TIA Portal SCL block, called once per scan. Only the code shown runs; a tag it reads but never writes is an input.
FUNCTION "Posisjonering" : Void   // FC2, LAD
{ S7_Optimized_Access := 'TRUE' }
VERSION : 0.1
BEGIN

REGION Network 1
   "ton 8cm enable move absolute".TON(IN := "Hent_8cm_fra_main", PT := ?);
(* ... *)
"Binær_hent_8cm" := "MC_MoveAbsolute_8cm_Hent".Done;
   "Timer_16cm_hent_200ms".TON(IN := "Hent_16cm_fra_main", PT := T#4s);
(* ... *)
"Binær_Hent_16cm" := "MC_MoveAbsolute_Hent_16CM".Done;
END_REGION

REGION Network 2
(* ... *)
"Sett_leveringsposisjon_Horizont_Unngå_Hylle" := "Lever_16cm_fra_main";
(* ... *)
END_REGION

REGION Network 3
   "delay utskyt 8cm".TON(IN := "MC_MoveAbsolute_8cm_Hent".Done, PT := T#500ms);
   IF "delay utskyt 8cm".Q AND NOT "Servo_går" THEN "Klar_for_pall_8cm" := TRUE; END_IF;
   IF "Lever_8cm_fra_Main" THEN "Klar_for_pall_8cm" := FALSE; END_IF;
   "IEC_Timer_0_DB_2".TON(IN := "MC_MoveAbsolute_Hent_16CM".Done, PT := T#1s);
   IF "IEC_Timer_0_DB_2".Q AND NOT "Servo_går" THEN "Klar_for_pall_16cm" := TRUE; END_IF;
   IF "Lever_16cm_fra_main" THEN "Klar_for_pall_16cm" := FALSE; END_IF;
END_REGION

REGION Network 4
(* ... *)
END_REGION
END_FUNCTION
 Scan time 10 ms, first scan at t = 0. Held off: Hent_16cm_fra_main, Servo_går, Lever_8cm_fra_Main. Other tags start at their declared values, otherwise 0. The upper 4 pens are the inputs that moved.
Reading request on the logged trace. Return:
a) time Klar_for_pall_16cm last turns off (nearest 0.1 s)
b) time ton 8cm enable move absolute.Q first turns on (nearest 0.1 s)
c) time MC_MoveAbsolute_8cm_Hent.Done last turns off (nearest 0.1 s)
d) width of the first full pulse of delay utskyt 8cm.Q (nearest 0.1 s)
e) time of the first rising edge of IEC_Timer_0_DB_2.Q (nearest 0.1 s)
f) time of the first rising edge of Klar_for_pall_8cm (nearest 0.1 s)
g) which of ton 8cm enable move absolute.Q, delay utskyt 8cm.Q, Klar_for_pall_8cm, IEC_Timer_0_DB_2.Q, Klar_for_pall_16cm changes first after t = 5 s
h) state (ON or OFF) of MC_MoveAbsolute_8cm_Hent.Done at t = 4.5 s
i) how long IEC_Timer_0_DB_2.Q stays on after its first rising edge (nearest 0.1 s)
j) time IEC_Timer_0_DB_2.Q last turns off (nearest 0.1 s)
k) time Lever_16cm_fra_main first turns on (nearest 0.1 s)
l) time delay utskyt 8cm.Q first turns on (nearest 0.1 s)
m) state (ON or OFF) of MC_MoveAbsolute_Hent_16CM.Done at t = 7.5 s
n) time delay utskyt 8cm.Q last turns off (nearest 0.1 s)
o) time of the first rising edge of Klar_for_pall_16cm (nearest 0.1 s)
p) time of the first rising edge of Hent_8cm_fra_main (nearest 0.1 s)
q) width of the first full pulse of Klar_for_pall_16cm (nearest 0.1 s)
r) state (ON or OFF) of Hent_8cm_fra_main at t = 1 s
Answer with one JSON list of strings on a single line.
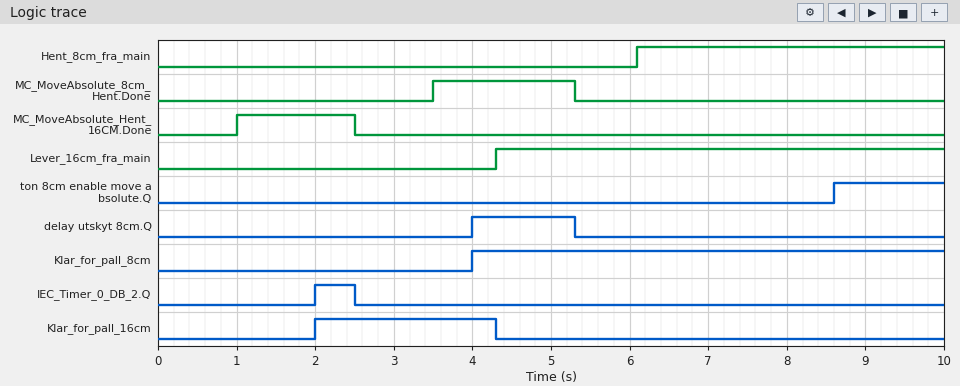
["4.3 s", "8.6 s", "5.3 s", "1.3 s", "2.0 s", "4.0 s", "delay utskyt 8cm.Q", "ON", "0.5 s", "2.5 s", "4.3 s", "4.0 s", "OFF", "5.3 s", "2.0 s", "6.1 s", "2.3 s", "OFF"]
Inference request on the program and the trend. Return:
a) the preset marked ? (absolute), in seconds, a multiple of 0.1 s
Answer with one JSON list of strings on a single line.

["2.5 s"]
